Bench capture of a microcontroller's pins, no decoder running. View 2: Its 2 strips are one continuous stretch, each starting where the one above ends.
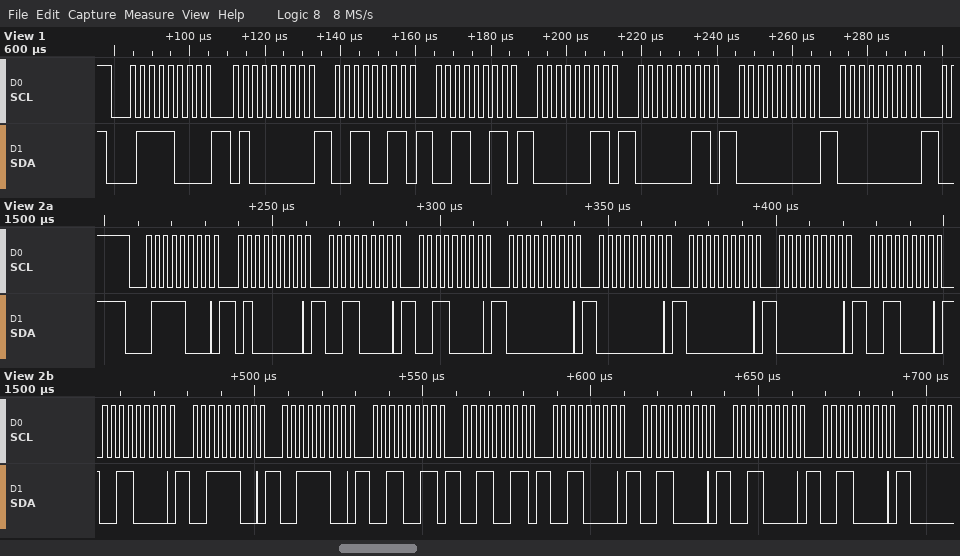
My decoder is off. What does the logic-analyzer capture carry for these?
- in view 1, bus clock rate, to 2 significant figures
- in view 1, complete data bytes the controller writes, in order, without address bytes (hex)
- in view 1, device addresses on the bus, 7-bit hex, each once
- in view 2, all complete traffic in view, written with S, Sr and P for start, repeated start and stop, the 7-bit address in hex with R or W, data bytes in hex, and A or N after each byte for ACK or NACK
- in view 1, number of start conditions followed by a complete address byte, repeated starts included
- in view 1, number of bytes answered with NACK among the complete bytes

400 kHz
40 33 33 03 03 00 00
0x3C
S 3CW A 40 A 30 A 30 A 00 A 00 A 00 A 00 A 30 A 30 A 3C A 3C A 33 A 33 A 30 A 30 A 30 A 30 A
1
0
